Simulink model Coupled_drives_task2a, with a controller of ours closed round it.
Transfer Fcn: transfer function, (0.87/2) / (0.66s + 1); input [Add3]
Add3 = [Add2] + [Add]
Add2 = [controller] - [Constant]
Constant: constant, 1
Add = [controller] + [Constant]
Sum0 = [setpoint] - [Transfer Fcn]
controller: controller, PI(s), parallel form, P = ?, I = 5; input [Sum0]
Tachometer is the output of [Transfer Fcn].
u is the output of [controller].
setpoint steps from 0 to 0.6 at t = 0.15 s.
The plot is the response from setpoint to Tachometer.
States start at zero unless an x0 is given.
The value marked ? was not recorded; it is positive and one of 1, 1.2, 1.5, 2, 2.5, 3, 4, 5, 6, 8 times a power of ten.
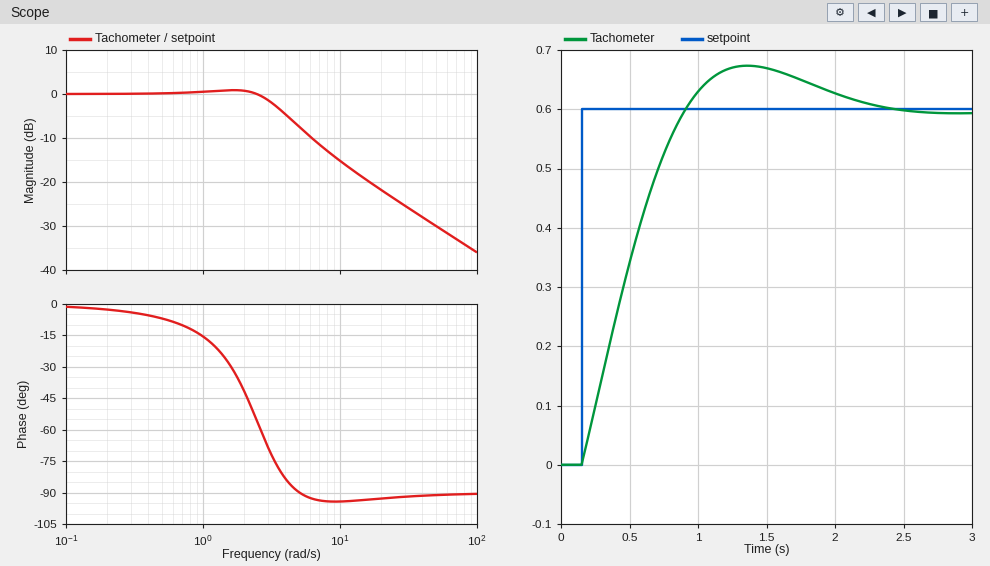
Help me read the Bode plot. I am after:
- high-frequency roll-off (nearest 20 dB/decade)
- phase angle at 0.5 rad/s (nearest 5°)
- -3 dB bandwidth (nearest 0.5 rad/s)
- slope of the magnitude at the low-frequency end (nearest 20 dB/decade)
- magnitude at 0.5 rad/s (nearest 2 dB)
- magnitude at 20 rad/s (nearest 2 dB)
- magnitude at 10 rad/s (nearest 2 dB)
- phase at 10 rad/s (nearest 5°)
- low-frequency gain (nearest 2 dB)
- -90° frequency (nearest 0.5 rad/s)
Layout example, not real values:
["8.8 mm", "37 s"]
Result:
["-20 dB/decade", "-5°", "3.5 rad/s", "0 dB/decade", "0 dB", "-22 dB", "-16 dB", "-95°", "0 dB", "5.0 rad/s"]
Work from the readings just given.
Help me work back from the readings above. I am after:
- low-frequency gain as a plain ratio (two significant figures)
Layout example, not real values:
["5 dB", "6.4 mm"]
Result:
["1.0"]
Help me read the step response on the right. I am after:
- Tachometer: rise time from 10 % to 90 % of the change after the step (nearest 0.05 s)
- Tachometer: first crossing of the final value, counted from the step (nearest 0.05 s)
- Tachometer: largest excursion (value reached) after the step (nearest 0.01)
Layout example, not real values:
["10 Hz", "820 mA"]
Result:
["0.55 s", "0.75 s", "0.67"]
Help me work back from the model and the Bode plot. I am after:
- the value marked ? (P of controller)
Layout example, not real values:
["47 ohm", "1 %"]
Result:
["1.2"]
